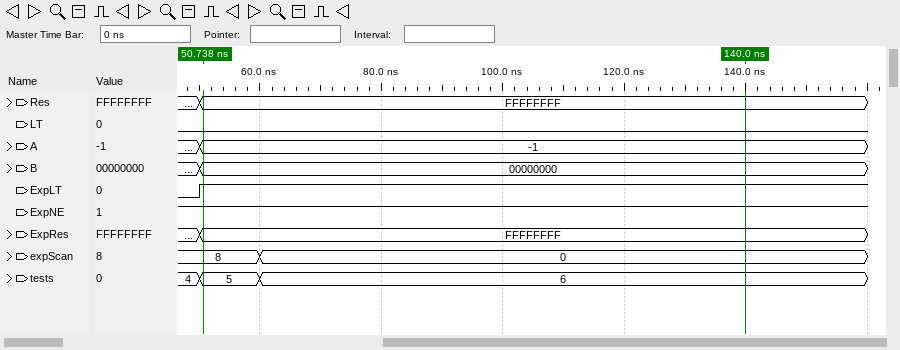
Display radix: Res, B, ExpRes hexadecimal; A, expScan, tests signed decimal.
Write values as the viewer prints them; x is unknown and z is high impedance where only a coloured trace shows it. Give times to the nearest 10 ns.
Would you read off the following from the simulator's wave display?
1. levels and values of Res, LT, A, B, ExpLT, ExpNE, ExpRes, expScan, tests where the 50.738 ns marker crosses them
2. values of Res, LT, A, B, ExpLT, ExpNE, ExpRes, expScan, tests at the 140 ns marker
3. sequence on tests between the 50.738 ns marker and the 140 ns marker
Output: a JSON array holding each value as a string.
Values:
["Res=FFFFFFFF, LT=0, A=-1, B=00000000, ExpLT=1, ExpNE=1, ExpRes=FFFFFFFF, expScan=8, tests=5", "Res=FFFFFFFF, LT=0, A=-1, B=00000000, ExpLT=1, ExpNE=1, ExpRes=FFFFFFFF, expScan=0, tests=6", "5, 6"]
